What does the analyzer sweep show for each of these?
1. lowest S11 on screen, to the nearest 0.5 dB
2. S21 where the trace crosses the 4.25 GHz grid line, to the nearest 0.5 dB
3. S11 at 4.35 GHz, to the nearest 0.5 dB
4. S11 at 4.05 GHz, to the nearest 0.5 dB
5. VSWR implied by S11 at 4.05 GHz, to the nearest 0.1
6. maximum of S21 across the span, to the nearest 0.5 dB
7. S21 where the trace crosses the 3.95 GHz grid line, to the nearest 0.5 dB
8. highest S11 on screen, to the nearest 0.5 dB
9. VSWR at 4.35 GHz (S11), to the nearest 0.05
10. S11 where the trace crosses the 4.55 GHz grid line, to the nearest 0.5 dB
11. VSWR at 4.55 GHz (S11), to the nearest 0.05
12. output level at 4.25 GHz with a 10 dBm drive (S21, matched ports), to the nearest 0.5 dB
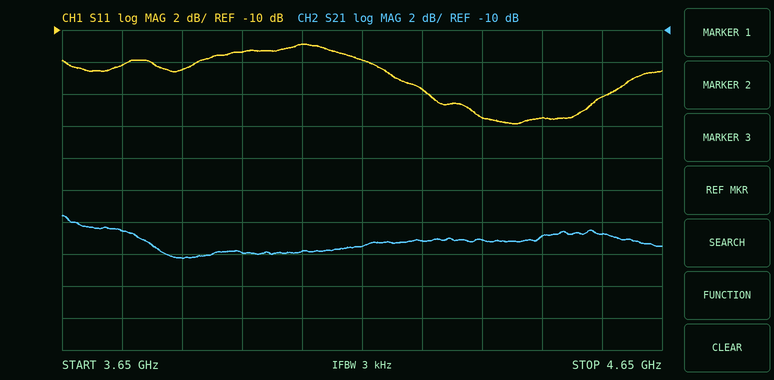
-16.0 dB
-23.0 dB
-15.5 dB
-11.0 dB
1.8
-21.5 dB
-24.0 dB
-11.0 dB
1.40
-14.0 dB
1.50
-13.0 dBm
